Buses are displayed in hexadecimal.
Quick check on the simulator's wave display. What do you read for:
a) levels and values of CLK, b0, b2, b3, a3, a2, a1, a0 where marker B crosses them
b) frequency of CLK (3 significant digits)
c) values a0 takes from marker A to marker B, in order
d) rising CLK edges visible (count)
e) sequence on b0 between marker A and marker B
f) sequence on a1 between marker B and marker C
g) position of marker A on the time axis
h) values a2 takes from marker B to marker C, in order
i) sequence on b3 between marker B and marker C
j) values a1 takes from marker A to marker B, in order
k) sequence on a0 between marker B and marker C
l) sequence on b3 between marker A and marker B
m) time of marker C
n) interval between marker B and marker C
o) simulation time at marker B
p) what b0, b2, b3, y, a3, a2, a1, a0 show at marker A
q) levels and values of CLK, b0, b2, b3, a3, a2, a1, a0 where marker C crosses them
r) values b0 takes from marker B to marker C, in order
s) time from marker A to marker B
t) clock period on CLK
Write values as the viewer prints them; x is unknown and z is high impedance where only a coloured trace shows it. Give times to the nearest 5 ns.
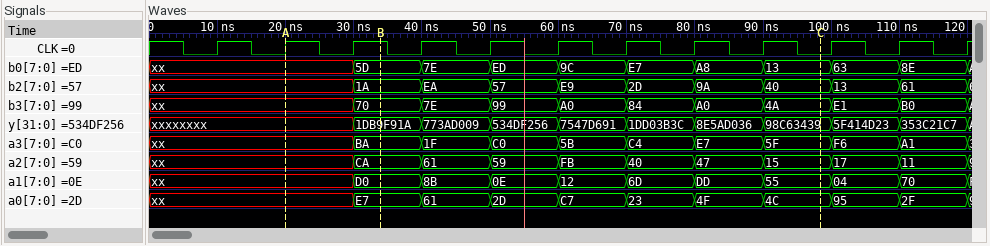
CLK=1, b0=5D, b2=1A, b3=70, a3=BA, a2=CA, a1=D0, a0=E7
100 MHz
xx, E7
12
xx, 5D
D0, 8B, 0E, 12, 6D, DD, 55
20 ns
CA, 61, 59, FB, 40, 47, 15
70, 7E, 99, A0, 84, A0, 4A
xx, D0
E7, 61, 2D, C7, 23, 4F, 4C
xx, 70
100 ns
65 ns
35 ns
b0=xx, b2=xx, b3=xx, y=xxxxxxxx, a3=xx, a2=xx, a1=xx, a0=xx
CLK=0, b0=13, b2=40, b3=4A, a3=5F, a2=15, a1=55, a0=4C
5D, 7E, ED, 9C, E7, A8, 13
15 ns
10 ns
